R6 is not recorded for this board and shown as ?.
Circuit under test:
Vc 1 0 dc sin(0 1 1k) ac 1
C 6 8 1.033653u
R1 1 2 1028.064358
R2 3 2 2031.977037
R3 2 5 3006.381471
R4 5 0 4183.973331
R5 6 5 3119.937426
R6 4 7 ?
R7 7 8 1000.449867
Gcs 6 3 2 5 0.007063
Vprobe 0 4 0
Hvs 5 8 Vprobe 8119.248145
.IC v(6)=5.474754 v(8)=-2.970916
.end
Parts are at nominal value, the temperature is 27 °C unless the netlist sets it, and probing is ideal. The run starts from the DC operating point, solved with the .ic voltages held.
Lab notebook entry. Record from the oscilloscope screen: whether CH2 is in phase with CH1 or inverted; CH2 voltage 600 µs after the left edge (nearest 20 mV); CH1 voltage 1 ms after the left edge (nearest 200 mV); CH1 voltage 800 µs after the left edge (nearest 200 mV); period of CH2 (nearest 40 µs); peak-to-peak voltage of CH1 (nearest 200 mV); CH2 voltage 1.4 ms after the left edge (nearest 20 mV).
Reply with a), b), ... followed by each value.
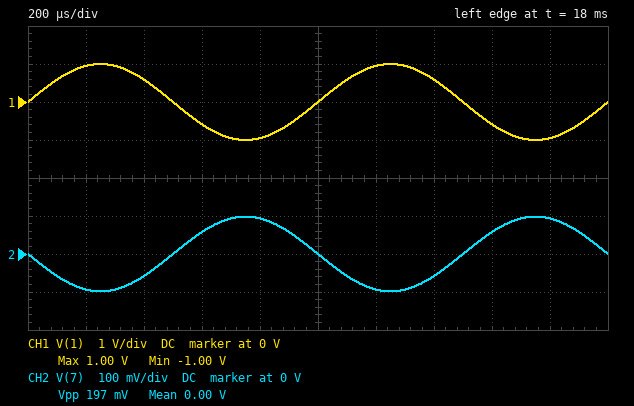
a) inverted
b) 60 mV
c) 0 V
d) -1.0 V
e) 1.00 ms
f) 2.0 V
g) -60 mV
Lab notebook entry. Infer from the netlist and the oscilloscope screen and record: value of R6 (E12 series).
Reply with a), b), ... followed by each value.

a) 680 Ω
